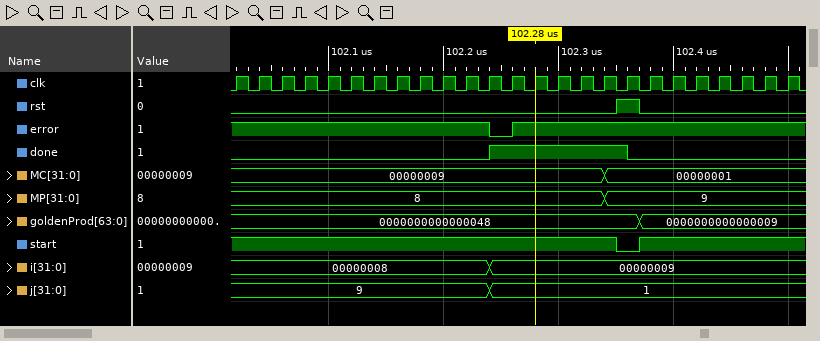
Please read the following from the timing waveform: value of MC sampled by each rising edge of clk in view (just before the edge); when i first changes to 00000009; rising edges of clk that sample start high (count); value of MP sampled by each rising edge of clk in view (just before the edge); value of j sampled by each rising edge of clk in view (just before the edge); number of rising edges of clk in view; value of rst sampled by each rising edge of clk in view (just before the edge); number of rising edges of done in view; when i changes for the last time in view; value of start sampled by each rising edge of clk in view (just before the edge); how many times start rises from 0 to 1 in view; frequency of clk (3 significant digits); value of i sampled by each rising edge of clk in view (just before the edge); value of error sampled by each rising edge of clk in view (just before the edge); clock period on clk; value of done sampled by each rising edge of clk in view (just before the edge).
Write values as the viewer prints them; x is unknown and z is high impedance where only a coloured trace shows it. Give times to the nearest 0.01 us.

00000009, 00000009, 00000009, 00000009, 00000009, 00000009, 00000009, 00000009, 00000009, 00000009, 00000009, 00000009, 00000009, 00000009, 00000009, 00000009, 00000009, 00000001, 00000001, 00000001, 00000001, 00000001, 00000001, 00000001, 00000001
102.24 us
24
8, 8, 8, 8, 8, 8, 8, 8, 8, 8, 8, 8, 8, 8, 8, 8, 8, 9, 9, 9, 9, 9, 9, 9, 9
9, 9, 9, 9, 9, 9, 9, 9, 9, 9, 9, 9, 1, 1, 1, 1, 1, 1, 1, 1, 1, 1, 1, 1, 1
25
0 0 0 0 0 0 0 0 0 0 0 0 0 0 0 0 0 1 0 0 0 0 0 0 0
1
102.24 us
1 1 1 1 1 1 1 1 1 1 1 1 1 1 1 1 1 0 1 1 1 1 1 1 1
1
50.0 MHz
00000008, 00000008, 00000008, 00000008, 00000008, 00000008, 00000008, 00000008, 00000008, 00000008, 00000008, 00000008, 00000009, 00000009, 00000009, 00000009, 00000009, 00000009, 00000009, 00000009, 00000009, 00000009, 00000009, 00000009, 00000009
1 1 1 1 1 1 1 1 1 1 1 1 0 1 1 1 1 1 1 1 1 1 1 1 1
0.02 us
0 0 0 0 0 0 0 0 0 0 0 0 1 1 1 1 1 1 0 0 0 0 0 0 0
